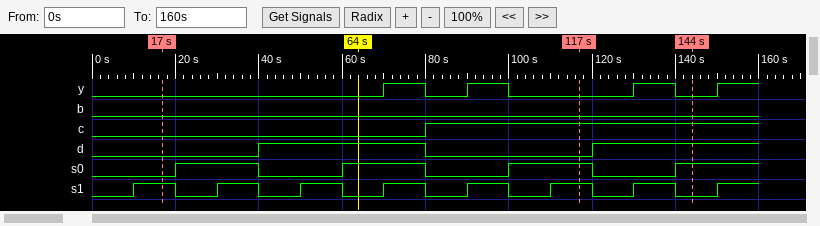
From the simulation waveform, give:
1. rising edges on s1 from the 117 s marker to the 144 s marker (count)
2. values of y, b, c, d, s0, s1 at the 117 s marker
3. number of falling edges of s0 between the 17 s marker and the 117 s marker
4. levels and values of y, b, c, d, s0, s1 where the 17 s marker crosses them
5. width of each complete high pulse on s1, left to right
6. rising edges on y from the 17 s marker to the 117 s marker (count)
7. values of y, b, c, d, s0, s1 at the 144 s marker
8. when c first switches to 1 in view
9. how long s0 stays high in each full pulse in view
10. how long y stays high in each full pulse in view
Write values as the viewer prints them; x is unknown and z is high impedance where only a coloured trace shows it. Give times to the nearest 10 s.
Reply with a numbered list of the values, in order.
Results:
1. 1
2. y=0, b=0, c=1, d=0, s0=1, s1=1
3. 2
4. y=0, b=0, c=0, d=0, s0=0, s1=1
5. 10 s, 10 s, 10 s, 10 s, 10 s, 10 s, 10 s
6. 2
7. y=0, b=0, c=1, d=1, s0=1, s1=0
8. 80 s
9. 20 s, 20 s, 20 s
10. 10 s, 10 s, 10 s
